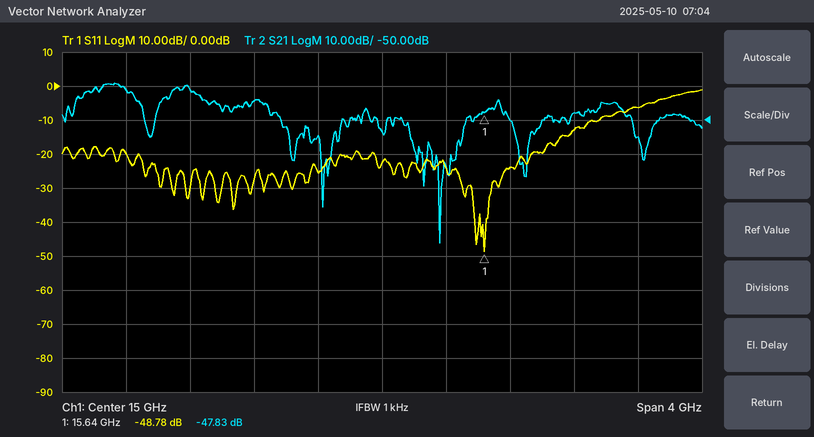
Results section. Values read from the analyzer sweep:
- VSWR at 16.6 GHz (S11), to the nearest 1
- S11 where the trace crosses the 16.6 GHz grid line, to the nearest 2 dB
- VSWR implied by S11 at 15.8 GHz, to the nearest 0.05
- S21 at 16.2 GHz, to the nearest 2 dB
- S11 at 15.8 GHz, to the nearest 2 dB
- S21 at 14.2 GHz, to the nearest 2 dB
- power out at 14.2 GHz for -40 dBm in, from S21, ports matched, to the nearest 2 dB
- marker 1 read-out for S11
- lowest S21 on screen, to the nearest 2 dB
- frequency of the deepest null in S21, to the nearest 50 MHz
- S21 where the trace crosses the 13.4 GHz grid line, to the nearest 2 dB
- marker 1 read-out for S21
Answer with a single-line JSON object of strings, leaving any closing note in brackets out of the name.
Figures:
{"VSWR at 16.6 GHz (S11), to the nearest 1": "3", "S11 where the trace crosses the 16.6 GHz grid line, to the nearest 2 dB": "-6 dB", "VSWR implied by S11 at 15.8 GHz, to the nearest 0.05": "1.15", "S21 at 16.2 GHz, to the nearest 2 dB": "-48 dB", "S11 at 15.8 GHz, to the nearest 2 dB": "-24 dB", "S21 at 14.2 GHz, to the nearest 2 dB": "-44 dB", "power out at 14.2 GHz for -40 dBm in, from S21, ports matched, to the nearest 2 dB": "-84 dBm", "marker 1 read-out for S11": "-48.78 dB", "lowest S21 on screen, to the nearest 2 dB": "-86 dB", "frequency of the deepest null in S21, to the nearest 50 MHz": "15.35 GHz", "S21 where the trace crosses the 13.4 GHz grid line, to the nearest 2 dB": "-42 dB", "marker 1 read-out for S21": "-47.83 dB"}
